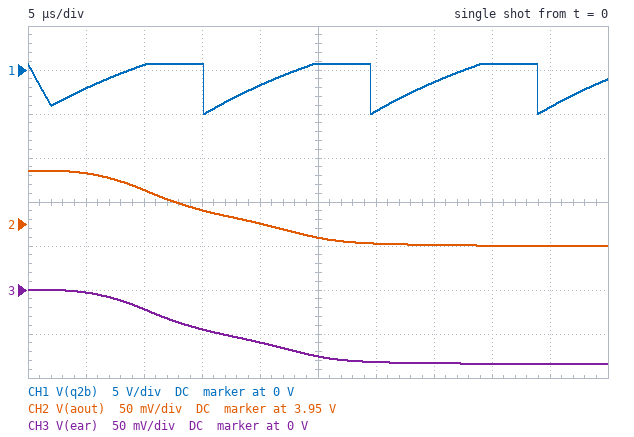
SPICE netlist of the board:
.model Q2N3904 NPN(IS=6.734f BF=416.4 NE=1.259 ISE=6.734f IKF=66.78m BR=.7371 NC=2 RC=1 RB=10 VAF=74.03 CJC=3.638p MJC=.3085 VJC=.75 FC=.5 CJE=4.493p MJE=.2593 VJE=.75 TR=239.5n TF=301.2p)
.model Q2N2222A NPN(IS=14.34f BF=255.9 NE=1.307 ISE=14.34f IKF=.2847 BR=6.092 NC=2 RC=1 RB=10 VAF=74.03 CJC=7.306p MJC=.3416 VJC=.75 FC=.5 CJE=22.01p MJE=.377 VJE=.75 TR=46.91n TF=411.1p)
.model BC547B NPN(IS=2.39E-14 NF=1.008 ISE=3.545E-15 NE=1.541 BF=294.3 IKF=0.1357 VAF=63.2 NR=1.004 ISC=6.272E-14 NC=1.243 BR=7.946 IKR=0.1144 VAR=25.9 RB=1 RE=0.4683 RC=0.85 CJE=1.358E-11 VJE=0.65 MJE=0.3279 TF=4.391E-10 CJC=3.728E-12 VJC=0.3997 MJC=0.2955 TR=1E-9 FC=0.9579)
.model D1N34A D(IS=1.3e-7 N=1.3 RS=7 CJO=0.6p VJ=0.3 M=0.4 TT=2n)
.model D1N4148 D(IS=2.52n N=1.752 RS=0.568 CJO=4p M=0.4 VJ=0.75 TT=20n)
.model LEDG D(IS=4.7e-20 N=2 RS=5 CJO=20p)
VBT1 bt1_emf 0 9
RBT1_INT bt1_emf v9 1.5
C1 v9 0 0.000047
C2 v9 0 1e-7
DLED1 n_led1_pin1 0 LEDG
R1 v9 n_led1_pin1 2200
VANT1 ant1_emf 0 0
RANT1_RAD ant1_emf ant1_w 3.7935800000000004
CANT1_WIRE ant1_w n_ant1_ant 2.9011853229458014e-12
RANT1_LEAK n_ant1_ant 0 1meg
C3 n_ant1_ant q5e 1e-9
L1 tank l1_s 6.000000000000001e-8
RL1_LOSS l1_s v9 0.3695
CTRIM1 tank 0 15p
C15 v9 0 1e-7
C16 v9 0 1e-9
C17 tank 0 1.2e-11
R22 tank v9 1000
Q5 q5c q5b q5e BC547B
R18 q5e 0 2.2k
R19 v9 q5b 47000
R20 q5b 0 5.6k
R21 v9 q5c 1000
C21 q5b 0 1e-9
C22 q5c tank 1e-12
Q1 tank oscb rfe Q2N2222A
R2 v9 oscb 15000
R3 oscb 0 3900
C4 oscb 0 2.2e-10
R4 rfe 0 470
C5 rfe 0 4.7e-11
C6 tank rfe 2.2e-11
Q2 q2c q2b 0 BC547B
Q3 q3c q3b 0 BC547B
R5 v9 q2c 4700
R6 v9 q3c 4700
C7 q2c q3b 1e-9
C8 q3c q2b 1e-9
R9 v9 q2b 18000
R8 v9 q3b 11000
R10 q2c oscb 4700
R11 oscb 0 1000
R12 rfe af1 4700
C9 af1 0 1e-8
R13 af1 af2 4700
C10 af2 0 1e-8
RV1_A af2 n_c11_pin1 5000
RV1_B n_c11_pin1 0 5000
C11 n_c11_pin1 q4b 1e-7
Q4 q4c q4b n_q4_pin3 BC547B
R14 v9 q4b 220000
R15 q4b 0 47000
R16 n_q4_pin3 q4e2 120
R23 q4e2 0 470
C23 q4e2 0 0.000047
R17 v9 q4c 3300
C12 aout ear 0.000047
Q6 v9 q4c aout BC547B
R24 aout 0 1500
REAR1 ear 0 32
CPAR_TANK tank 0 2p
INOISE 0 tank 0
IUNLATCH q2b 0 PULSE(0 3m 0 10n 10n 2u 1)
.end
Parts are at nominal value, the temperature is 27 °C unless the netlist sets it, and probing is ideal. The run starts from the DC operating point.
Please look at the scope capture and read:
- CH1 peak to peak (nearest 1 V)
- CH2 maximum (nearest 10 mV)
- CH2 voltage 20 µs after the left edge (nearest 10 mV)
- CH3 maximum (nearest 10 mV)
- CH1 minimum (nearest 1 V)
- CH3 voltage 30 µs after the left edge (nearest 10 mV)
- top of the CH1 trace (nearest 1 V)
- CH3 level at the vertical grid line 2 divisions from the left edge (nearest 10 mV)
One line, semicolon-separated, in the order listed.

6 V; 4.01 V; 3.95 V; 0 V; -5 V; -80 mV; 1 V; -20 mV
